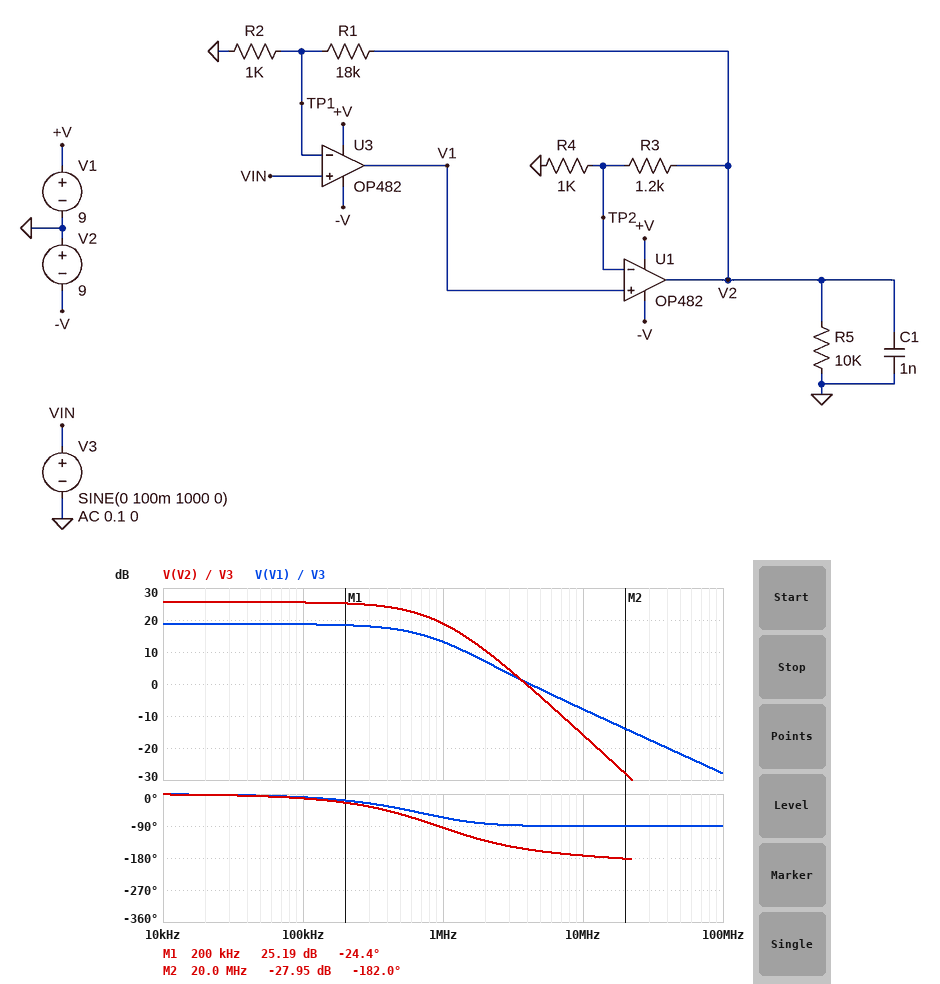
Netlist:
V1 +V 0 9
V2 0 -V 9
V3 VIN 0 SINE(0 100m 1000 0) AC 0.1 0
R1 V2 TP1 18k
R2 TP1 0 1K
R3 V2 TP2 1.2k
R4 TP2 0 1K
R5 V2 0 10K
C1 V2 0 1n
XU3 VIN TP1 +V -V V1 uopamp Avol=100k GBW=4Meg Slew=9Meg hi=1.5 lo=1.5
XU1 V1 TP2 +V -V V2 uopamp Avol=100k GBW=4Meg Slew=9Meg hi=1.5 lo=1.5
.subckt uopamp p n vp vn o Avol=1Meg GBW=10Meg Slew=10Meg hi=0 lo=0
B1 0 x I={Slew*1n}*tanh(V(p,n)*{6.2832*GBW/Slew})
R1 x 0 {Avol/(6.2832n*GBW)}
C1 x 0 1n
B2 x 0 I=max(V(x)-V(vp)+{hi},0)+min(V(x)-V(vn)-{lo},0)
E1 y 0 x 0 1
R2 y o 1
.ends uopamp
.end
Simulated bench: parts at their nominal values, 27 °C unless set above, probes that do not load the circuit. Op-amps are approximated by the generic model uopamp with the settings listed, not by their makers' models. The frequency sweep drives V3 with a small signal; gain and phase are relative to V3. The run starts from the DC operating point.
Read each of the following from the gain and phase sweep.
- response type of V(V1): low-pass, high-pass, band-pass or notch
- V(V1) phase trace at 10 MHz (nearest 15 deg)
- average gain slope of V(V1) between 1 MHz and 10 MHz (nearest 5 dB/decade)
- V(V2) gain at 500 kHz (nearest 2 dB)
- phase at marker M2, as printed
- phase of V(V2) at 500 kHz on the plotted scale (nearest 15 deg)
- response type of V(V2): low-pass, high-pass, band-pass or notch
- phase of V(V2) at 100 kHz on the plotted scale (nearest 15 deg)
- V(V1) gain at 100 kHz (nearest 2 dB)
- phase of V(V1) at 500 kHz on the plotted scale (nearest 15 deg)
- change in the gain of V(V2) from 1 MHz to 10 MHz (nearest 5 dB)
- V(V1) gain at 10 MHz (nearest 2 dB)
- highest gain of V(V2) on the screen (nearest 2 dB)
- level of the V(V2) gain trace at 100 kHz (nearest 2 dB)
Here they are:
low-pass
-90 deg
-20 dB/decade
24 dB
-182.0 deg
-60 deg
low-pass
-15 deg
18 dB
-45 deg
-35 dB
-8 dB
26 dB
26 dB
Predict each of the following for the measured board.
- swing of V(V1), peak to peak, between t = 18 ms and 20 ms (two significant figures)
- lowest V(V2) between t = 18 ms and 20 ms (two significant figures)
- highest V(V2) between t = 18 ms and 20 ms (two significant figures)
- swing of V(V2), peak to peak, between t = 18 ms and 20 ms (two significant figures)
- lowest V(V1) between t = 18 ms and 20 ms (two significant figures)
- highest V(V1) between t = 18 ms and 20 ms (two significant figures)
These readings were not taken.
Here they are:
1.7 V
-1.9 V
1.9 V
3.8 V
-860 mV
860 mV
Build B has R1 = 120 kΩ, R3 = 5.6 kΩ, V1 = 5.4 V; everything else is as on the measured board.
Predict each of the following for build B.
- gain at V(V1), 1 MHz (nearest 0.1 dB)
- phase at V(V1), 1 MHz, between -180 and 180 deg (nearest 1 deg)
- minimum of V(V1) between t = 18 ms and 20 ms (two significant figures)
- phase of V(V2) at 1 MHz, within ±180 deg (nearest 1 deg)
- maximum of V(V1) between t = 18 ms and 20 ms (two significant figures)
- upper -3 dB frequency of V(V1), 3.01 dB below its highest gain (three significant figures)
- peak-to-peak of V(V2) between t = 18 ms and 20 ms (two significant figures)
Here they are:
12.9 dB
-86 deg
-7.5 V
-145 deg
3.9 V
359 kHz
11 V
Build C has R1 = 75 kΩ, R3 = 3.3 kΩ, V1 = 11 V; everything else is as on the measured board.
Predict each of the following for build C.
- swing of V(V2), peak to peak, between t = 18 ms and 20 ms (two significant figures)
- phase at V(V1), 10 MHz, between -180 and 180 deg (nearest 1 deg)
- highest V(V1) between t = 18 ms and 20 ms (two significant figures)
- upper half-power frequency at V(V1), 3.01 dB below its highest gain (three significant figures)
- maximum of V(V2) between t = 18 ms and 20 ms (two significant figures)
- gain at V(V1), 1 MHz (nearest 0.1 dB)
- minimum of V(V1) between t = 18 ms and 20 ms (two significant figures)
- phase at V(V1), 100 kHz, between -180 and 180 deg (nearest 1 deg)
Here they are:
15 V
-90 deg
1.8 V
317 kHz
7.6 V
13.0 dB
-2.8 V
-19 deg
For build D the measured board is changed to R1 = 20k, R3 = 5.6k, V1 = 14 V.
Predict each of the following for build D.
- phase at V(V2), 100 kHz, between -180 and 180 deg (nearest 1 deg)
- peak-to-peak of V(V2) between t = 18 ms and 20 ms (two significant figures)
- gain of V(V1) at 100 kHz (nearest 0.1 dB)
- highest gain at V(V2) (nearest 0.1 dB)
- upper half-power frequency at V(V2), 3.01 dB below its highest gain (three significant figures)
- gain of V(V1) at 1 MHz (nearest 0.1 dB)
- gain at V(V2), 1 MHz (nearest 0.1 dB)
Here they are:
-5 deg
4.2 V
10.3 dB
30.2 dB
1.04 MHz
17.2 dB
27.9 dB
